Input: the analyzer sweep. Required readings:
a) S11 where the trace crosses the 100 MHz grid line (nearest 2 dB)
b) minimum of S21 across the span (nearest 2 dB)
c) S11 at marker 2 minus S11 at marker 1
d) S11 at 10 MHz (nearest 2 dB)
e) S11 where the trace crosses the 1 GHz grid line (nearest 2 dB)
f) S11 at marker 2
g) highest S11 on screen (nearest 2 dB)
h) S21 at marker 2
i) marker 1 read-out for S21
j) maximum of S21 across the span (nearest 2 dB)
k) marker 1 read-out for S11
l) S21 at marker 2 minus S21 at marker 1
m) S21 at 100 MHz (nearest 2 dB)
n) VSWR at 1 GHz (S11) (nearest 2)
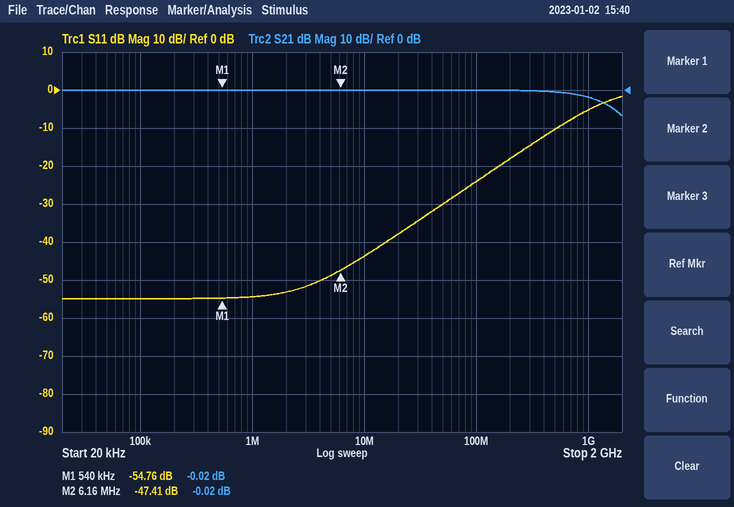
-24 dB
-6 dB
7.35 dB
-44 dB
-6 dB
-47.41 dB
-2 dB
-0.02 dB
-0.02 dB
0 dB
-54.76 dB
0.00 dB
0 dB
4
